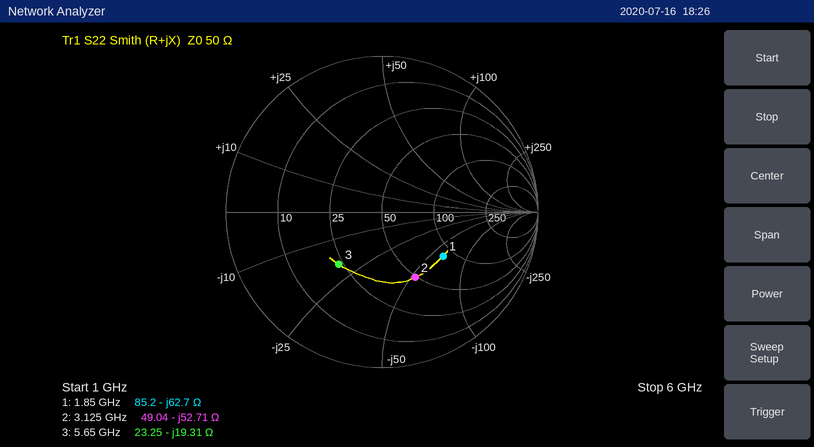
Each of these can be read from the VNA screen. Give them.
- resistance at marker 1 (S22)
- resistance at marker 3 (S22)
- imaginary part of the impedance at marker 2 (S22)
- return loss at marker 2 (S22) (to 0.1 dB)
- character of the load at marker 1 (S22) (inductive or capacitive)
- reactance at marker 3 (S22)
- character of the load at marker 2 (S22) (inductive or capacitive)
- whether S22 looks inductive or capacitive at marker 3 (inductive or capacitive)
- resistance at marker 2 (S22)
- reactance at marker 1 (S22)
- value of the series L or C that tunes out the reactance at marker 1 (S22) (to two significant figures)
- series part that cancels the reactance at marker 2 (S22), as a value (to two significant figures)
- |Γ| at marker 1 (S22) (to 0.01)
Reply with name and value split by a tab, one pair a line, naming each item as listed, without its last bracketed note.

resistance at marker 1	85.2 Ω
resistance at marker 3	23.25 Ω
imaginary part of the impedance at marker 2	-52.71 Ω
return loss at marker 2 (S22)	6.6 dB
character of the load at marker 1 (S22)	capacitive
reactance at marker 3	-19.31 Ω
character of the load at marker 2 (S22)	capacitive
whether S22 looks inductive or capacitive at marker 3	capacitive
resistance at marker 2	49.04 Ω
reactance at marker 1	-62.7 Ω
value of the series L or C that tunes out the reactance at marker 1 (S22)	5.4 nH
series part that cancels the reactance at marker 2 (S22), as a value	2.7 nH
|Γ| at marker 1 (S22)	0.48
